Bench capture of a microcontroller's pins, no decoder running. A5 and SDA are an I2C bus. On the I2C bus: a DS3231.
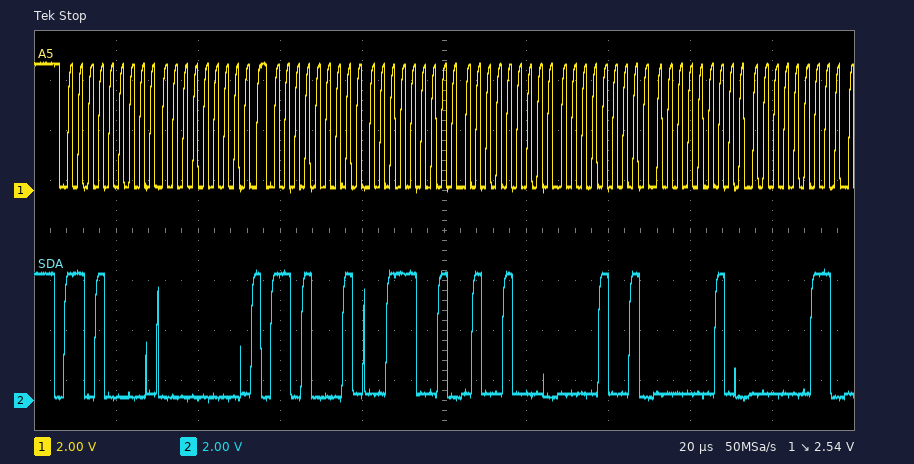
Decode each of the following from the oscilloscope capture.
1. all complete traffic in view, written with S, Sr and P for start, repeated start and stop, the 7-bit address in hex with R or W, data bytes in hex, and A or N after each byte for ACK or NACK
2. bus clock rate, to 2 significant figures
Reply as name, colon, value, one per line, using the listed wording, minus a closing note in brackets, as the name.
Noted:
all complete traffic in view, written with S, Sr and P for start, repeated start and stop, the 7-bit address in hex with R or W, data bytes in hex, and A or N after each byte for ACK or NACK: S 68W A 00 A Sr 68R A 39 A 48 A 09 A 02 A 03 A
bus clock rate, to 2 significant figures: 400 kHz
